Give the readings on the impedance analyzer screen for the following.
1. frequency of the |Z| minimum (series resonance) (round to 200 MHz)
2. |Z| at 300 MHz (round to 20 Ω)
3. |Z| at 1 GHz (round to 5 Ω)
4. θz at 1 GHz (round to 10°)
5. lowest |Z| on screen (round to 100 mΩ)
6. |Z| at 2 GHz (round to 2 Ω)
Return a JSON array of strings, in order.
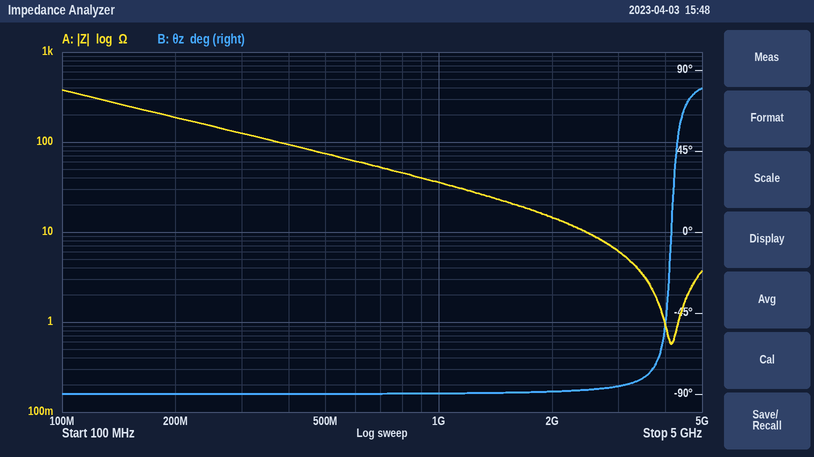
["4.2 GHz", "120 Ω", "35 Ω", "-90°", "600 mΩ", "14 Ω"]
